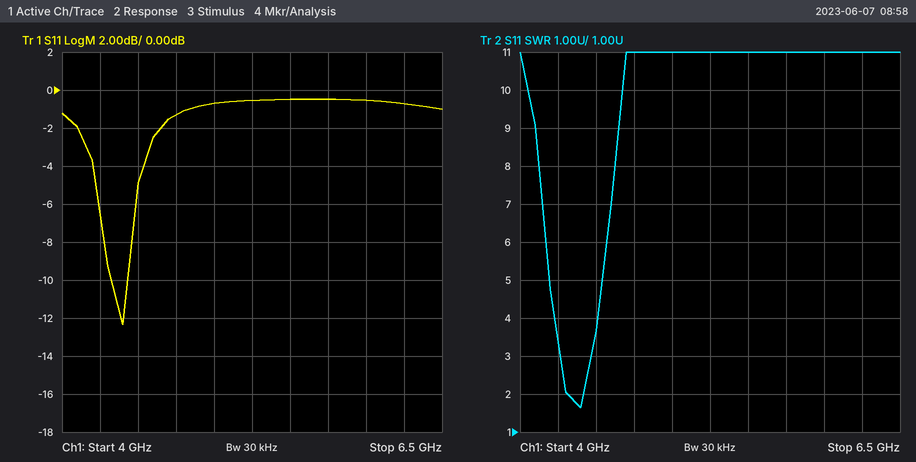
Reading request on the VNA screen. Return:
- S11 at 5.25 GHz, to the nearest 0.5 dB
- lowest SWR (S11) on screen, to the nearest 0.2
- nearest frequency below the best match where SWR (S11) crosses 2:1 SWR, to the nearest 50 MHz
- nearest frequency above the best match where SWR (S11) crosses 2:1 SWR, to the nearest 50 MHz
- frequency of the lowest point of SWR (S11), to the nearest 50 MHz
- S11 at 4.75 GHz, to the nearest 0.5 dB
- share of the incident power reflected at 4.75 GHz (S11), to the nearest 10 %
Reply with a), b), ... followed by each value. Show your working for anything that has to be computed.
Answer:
a) -0.5 dB
b) 1.6
c) 4.30 GHz
d) 4.40 GHz
e) 4.40 GHz
f) -1.5 dB
g) 10^(-1.5/10) ≈ 70.8 %, so 70 % to the nearest 10 %
